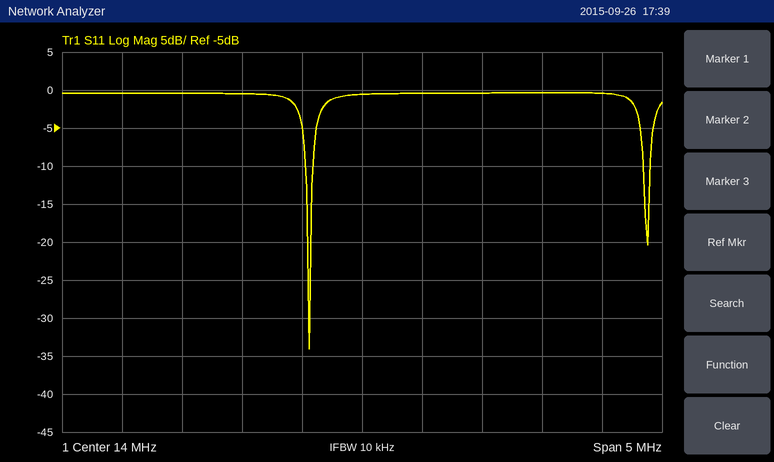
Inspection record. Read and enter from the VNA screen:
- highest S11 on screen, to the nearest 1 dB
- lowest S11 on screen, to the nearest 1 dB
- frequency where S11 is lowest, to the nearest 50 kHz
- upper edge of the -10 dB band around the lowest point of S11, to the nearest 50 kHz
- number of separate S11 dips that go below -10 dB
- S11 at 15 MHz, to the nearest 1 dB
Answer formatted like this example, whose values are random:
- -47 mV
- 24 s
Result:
- 0 dB
- -34 dB
- 13.55 MHz
- 13.60 MHz
- 2
- 0 dB
